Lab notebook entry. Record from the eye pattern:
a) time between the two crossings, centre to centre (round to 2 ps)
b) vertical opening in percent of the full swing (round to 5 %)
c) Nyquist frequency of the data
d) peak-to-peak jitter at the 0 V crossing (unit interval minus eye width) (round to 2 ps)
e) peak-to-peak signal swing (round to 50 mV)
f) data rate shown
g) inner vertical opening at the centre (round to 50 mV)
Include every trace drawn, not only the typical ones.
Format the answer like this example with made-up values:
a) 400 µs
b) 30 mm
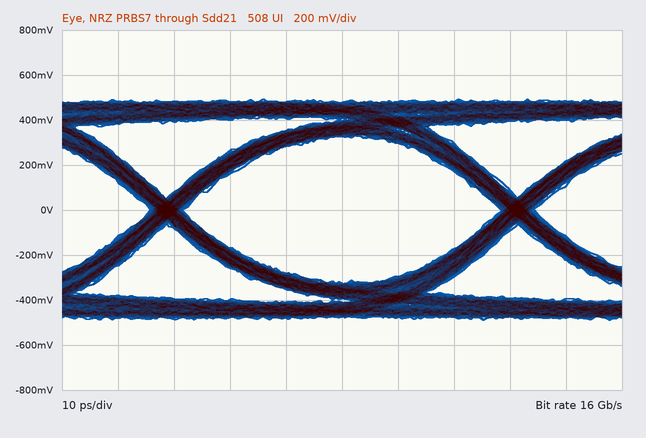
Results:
a) 62 ps
b) 65 %
c) 8 GHz
d) 6 ps
e) 1.00 V
f) 16 Gb/s
g) 650 mV
